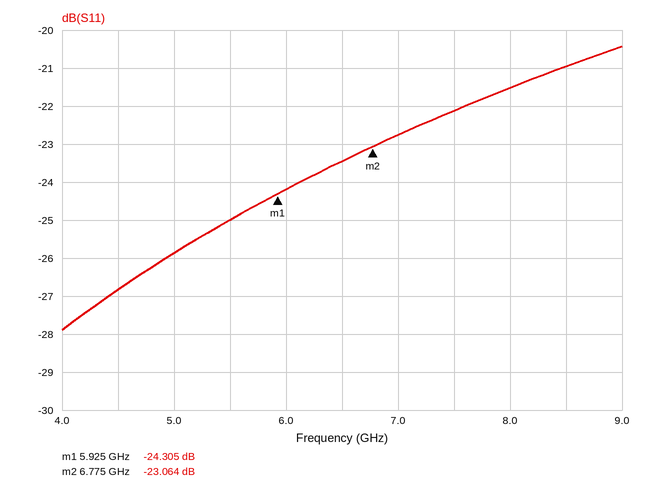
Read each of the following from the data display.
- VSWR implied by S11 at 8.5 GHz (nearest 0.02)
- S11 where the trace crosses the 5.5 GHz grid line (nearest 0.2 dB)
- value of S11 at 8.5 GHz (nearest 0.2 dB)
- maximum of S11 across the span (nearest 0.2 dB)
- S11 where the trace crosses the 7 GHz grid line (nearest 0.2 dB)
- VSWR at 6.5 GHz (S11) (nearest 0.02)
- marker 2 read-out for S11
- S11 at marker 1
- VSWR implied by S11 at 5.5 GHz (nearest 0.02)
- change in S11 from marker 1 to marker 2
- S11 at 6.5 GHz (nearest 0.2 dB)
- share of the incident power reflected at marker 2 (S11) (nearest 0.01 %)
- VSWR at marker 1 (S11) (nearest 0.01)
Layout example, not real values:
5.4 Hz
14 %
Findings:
1.20
-25.0 dB
-21.0 dB
-20.4 dB
-22.8 dB
1.14
-23.064 dB
-24.305 dB
1.12
1.241 dB
-23.4 dB
0.49 %
1.13
